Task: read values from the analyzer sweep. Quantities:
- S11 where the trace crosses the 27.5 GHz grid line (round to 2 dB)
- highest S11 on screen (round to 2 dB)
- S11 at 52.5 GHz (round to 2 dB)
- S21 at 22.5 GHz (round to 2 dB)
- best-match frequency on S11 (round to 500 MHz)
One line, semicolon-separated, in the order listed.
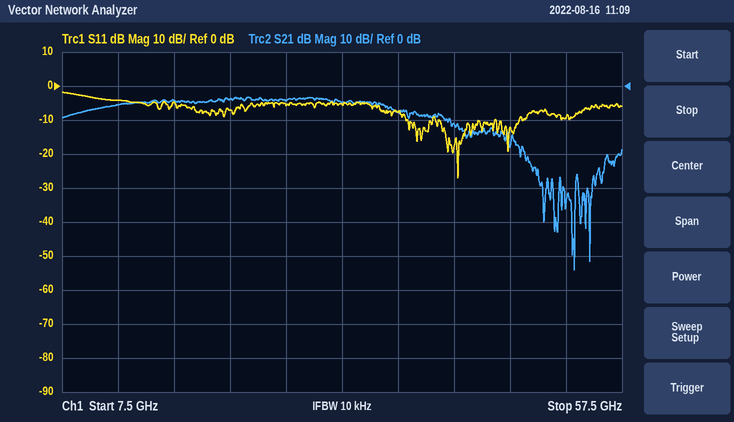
-6 dB; -2 dB; -10 dB; -4 dB; 43.0 GHz
